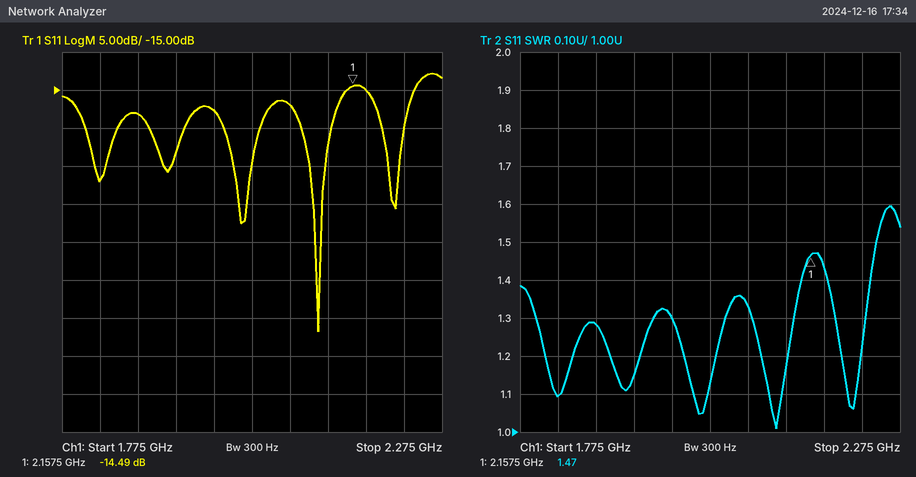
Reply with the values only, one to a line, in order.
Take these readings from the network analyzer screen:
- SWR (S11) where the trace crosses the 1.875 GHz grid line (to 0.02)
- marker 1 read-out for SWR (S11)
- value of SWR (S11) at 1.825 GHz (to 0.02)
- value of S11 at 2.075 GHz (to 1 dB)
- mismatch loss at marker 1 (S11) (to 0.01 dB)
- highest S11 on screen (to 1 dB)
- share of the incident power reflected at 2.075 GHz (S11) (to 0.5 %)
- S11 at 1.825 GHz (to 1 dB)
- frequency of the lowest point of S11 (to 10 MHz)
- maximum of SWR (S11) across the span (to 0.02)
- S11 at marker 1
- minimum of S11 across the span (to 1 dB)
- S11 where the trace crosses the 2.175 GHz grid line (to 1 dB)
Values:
1.28
1.47
1.10
-17 dB
0.16 dB
-13 dB
2.0 %
-27 dB
2.11 GHz
1.60
-14.49 dB
-47 dB
-15 dB
